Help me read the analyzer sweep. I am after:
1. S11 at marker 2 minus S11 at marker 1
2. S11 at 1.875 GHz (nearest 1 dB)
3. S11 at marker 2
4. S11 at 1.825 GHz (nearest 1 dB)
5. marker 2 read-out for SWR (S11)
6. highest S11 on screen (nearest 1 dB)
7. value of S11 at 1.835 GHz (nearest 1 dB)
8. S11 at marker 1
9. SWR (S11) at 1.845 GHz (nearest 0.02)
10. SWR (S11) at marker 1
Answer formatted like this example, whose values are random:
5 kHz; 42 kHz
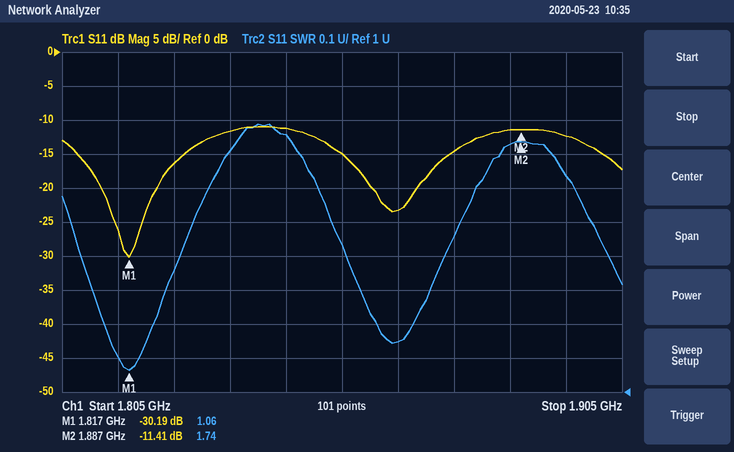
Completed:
18.78 dB; -15 dB; -11.41 dB; -16 dB; 1.74; -11 dB; -12 dB; -30.19 dB; 1.76; 1.06
